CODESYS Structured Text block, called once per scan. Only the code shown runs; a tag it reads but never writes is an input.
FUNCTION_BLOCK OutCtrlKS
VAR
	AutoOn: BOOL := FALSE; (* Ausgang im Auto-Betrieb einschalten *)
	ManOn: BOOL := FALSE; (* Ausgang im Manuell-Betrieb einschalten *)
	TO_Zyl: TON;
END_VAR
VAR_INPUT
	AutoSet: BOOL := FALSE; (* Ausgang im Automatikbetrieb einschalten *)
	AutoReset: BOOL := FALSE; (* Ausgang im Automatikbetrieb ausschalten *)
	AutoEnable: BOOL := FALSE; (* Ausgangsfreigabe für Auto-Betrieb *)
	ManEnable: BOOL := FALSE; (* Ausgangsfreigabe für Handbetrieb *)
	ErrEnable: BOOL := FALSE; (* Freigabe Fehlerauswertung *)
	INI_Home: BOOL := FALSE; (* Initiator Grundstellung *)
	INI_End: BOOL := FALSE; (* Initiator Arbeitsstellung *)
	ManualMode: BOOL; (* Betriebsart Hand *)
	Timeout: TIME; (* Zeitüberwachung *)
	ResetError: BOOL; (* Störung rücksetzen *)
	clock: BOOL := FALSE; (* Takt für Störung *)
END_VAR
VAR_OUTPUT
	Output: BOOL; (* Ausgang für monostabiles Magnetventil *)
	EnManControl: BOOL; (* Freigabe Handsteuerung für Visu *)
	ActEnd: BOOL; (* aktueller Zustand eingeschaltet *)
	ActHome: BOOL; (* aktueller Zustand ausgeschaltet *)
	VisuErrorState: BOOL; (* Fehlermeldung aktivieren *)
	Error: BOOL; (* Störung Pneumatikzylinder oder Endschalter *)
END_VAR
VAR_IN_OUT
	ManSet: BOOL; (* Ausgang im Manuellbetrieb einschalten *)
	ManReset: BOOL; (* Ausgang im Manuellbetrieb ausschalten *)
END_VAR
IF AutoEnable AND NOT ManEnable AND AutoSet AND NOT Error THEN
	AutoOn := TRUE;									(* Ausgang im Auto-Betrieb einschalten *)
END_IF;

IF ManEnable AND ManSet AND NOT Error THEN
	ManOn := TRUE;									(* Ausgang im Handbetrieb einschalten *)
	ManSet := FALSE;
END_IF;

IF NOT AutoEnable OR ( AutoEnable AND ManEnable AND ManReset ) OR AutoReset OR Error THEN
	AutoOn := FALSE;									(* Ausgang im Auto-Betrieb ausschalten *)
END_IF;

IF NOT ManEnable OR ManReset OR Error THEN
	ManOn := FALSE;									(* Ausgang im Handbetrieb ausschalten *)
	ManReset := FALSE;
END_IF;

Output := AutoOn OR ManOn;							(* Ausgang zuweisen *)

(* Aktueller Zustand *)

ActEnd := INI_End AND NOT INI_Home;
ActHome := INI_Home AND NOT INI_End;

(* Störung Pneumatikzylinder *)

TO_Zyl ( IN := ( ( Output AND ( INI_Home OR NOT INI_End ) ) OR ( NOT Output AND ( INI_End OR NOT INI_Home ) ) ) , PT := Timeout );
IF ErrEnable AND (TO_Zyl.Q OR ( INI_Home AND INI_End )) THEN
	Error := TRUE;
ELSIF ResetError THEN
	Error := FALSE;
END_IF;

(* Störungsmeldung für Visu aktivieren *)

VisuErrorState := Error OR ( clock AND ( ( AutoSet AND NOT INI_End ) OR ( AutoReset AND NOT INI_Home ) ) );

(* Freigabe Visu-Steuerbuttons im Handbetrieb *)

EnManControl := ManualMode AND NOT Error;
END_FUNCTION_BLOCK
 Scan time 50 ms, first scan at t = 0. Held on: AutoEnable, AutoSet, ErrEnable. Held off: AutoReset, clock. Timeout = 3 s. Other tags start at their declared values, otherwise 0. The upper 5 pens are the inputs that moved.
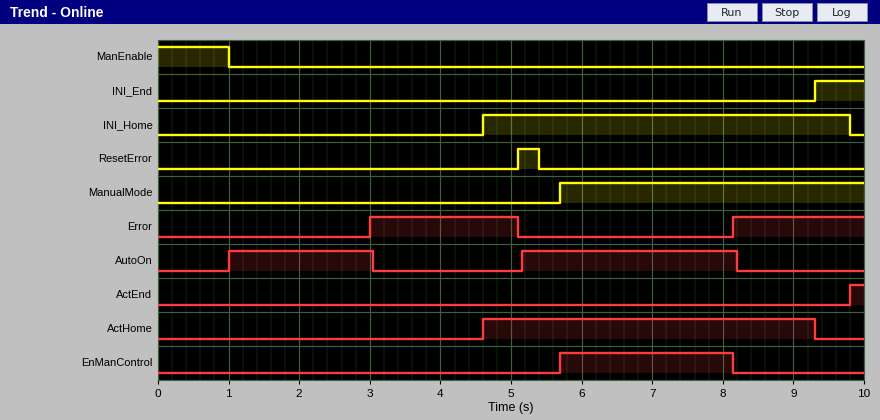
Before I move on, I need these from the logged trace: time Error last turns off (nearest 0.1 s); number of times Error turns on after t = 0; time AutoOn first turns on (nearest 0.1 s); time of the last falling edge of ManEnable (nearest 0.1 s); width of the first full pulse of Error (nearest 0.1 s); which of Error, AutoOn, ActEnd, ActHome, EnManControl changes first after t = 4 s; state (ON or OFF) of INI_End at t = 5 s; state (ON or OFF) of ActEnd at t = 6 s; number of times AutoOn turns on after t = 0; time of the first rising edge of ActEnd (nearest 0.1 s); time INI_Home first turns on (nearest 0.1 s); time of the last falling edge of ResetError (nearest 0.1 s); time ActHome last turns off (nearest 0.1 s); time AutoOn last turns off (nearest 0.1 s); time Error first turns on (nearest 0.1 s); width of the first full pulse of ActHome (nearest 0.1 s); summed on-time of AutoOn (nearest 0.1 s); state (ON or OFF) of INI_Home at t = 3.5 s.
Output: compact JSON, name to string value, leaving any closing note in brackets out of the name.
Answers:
{"time Error last turns off": "5.1 s", "number of times Error turns on after t = 0": "2", "time AutoOn first turns on": "1.0 s", "time of the last falling edge of ManEnable": "1.0 s", "width of the first full pulse of Error": "2.1 s", "which of Error, AutoOn, ActEnd, ActHome, EnManControl changes first after t = 4 s": "ActHome", "state (ON or OFF) of INI_End at t = 5 s": "OFF", "state (ON or OFF) of ActEnd at t = 6 s": "OFF", "number of times AutoOn turns on after t = 0": "2", "time of the first rising edge of ActEnd": "9.8 s", "time INI_Home first turns on": "4.6 s", "time of the last falling edge of ResetError": "5.4 s", "time ActHome last turns off": "9.3 s", "time AutoOn last turns off": "8.2 s", "time Error first turns on": "3.0 s", "width of the first full pulse of ActHome": "4.7 s", "summed on-time of AutoOn": "5.1 s", "state (ON or OFF) of INI_Home at t = 3.5 s": "OFF"}
